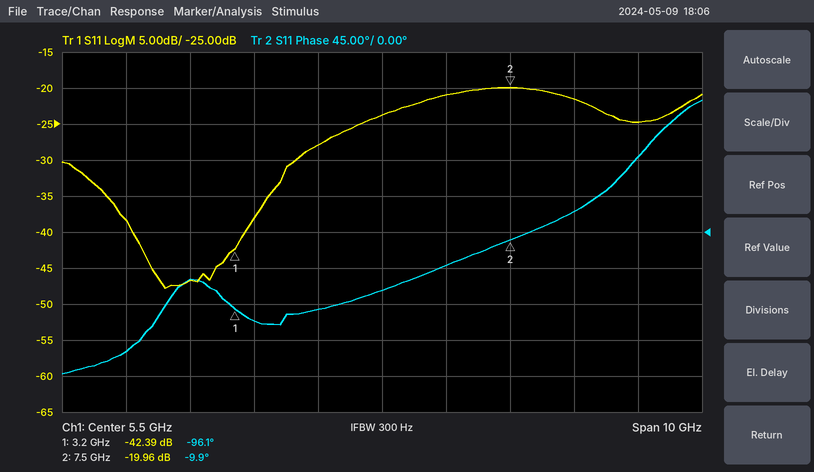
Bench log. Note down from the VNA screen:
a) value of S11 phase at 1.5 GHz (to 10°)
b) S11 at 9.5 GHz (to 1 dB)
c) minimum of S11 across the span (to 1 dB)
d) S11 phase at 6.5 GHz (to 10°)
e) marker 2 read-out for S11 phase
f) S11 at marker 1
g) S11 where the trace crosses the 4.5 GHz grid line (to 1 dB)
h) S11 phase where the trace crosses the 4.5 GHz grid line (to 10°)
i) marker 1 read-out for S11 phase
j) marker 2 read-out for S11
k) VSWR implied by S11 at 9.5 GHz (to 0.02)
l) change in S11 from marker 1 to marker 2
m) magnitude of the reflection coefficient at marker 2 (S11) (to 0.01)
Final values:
-150°
-25 dB
-48 dB
-40°
-9.9°
-42.39 dB
-28 dB
-100°
-96.1°
-19.96 dB
1.12
22.43 dB
0.10
